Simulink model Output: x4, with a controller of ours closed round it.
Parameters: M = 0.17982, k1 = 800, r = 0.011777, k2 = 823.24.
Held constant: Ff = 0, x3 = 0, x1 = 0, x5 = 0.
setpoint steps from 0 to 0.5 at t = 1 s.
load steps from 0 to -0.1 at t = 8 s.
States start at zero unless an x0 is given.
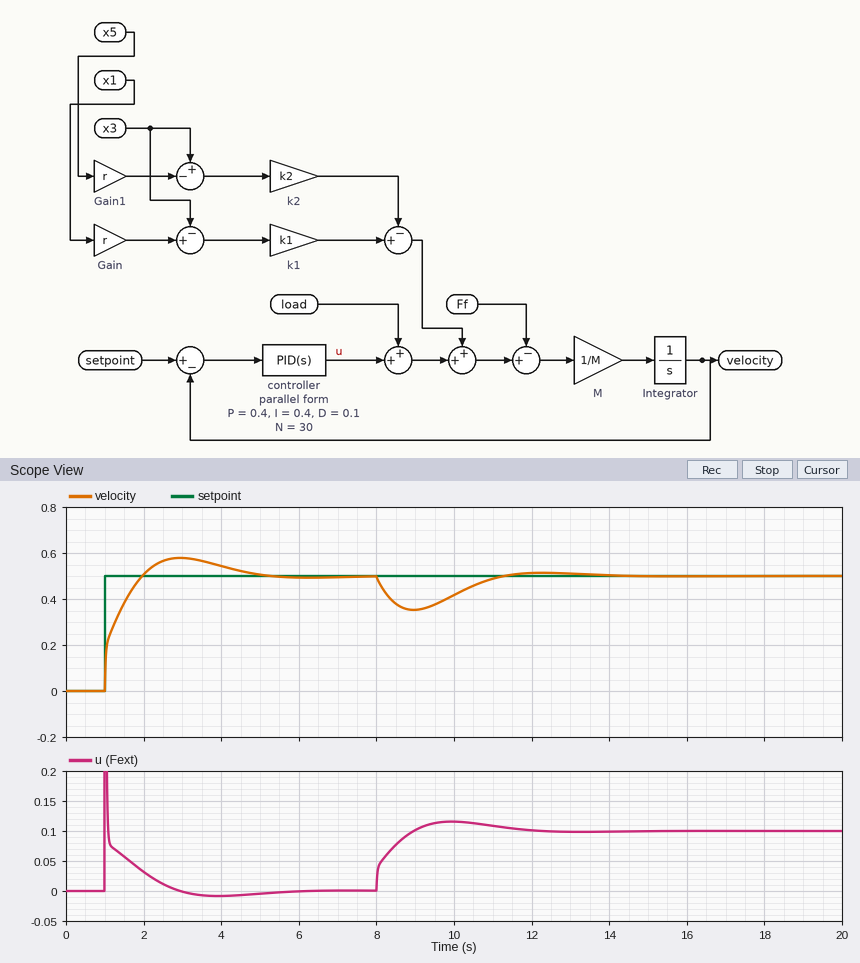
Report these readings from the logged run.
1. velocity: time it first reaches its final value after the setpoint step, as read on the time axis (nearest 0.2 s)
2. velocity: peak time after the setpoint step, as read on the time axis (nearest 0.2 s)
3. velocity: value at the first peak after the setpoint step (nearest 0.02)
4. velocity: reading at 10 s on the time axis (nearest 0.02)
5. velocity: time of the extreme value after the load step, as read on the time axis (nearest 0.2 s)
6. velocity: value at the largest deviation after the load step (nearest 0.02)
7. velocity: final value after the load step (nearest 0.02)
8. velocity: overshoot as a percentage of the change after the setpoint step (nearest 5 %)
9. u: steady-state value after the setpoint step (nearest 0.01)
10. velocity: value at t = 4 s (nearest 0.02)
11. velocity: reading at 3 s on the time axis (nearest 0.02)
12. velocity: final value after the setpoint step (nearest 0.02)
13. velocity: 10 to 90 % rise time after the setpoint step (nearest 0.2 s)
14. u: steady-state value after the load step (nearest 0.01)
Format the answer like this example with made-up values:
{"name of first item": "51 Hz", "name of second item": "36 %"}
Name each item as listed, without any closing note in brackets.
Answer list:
{"velocity: time it first reaches its final value after the setpoint step, as read on the time axis": "2.0 s", "velocity: peak time after the setpoint step, as read on the time axis": "3.0 s", "velocity: value at the first peak after the setpoint step": "0.58", "velocity: reading at 10 s on the time axis": "0.42", "velocity: time of the extreme value after the load step, as read on the time axis": "9.0 s", "velocity: value at the largest deviation after the load step": "0.36", "velocity: final value after the load step": "0.50", "velocity: overshoot as a percentage of the change after the setpoint step": "15 %", "u: steady-state value after the setpoint step": "0.00", "velocity: value at t = 4 s": "0.54", "velocity: reading at 3 s on the time axis": "0.58", "velocity: final value after the setpoint step": "0.50", "velocity: 10 to 90 % rise time after the setpoint step": "0.8 s", "u: steady-state value after the load step": "0.10"}
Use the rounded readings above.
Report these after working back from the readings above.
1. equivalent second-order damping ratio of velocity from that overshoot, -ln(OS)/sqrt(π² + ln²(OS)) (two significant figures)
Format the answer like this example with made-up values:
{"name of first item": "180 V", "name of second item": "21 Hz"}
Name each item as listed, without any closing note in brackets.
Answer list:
{"equivalent second-order damping ratio of velocity from that overshoot, -ln(OS)/sqrt(π² + ln²(OS))": "0.52"}
